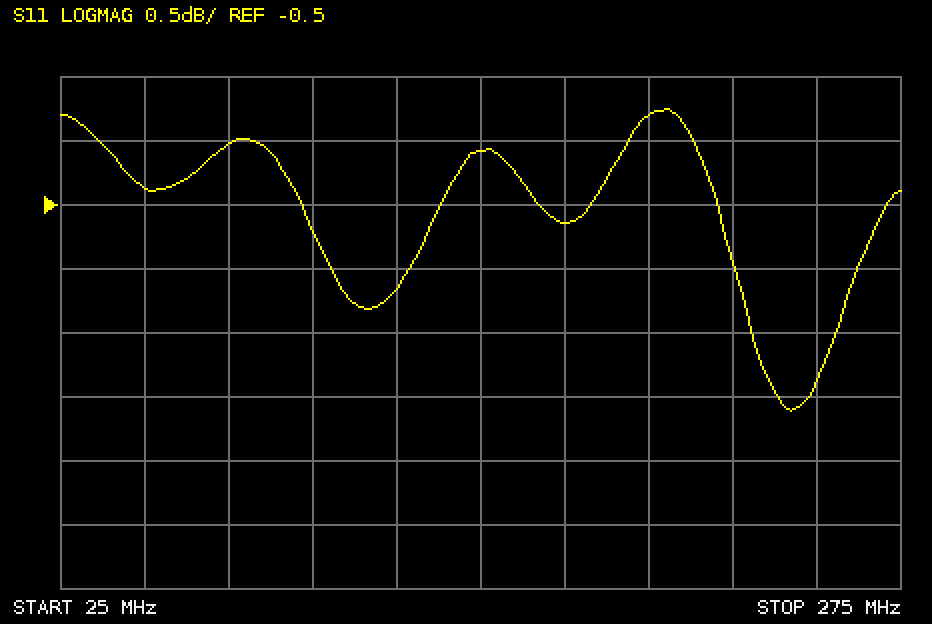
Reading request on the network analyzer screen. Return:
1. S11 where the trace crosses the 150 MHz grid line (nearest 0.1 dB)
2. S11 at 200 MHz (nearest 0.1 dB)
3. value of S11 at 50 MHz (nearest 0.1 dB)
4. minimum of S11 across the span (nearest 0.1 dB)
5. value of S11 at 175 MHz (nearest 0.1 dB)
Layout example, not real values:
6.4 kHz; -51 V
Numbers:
-0.1 dB; 0.2 dB; -0.4 dB; -2.1 dB; -0.6 dB
